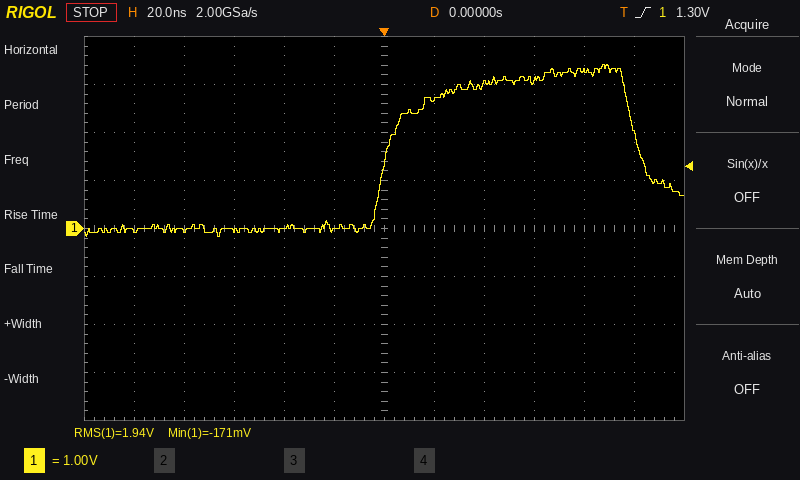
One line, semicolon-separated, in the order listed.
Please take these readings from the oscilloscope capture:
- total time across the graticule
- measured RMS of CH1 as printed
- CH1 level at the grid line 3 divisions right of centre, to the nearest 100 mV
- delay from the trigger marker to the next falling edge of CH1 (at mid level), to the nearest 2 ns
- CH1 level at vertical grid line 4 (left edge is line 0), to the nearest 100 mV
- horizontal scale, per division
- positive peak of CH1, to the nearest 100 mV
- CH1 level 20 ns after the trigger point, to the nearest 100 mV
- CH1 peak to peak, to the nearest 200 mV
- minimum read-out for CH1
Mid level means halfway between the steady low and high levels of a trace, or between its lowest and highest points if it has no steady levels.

240 ns; 1.94 V; 3.1 V; 102 ns; 0.0 V; 20 ns; 3.4 V; 2.7 V; 3.6 V; -171 mV
